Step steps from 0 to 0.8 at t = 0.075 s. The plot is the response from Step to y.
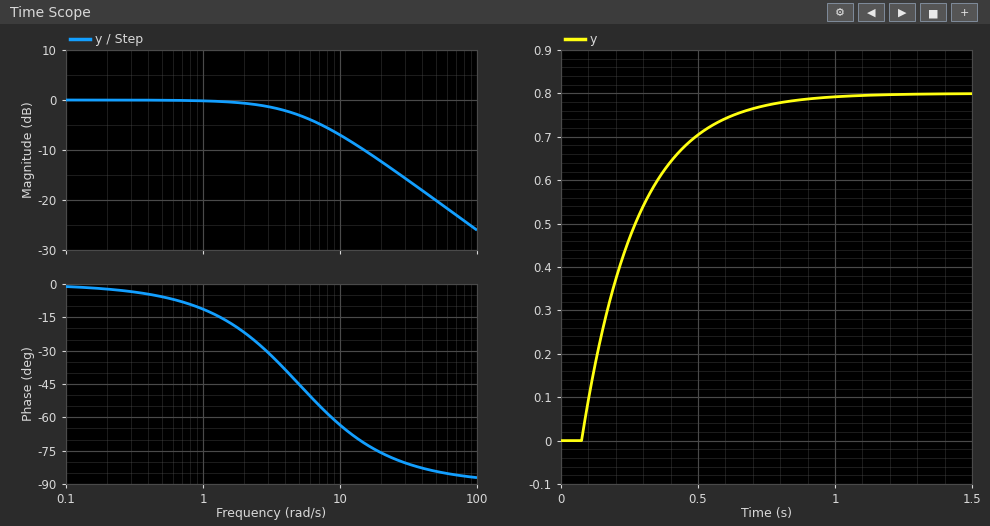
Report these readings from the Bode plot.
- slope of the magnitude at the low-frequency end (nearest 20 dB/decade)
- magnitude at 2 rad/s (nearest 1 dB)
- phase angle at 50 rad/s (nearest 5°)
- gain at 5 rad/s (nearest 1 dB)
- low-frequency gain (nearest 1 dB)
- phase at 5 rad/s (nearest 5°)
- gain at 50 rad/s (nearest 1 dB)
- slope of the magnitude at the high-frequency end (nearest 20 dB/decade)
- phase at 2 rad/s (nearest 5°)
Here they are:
0 dB/decade
-1 dB
-85°
-3 dB
0 dB
-45°
-20 dB
-20 dB/decade
-20°
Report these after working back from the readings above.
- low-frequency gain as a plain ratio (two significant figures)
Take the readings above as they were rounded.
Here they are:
1.0
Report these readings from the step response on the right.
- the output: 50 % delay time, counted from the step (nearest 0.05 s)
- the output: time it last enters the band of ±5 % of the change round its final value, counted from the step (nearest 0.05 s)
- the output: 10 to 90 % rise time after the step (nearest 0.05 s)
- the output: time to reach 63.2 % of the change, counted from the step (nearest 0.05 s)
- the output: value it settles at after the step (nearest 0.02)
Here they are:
0.15 s
0.60 s
0.45 s
0.20 s
0.80
